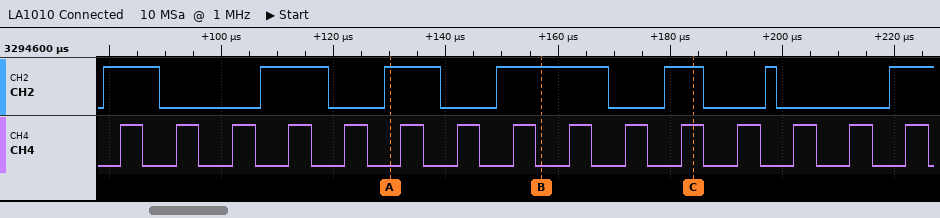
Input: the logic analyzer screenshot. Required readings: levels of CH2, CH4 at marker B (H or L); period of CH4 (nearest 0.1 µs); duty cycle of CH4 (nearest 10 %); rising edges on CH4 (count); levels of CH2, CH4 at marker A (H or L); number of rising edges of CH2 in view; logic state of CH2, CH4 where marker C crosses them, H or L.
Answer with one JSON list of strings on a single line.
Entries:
["CH2=H, CH4=L", "10 µs", "40 %", "15", "CH2=H, CH4=L", "7", "CH2=H, CH4=H"]
